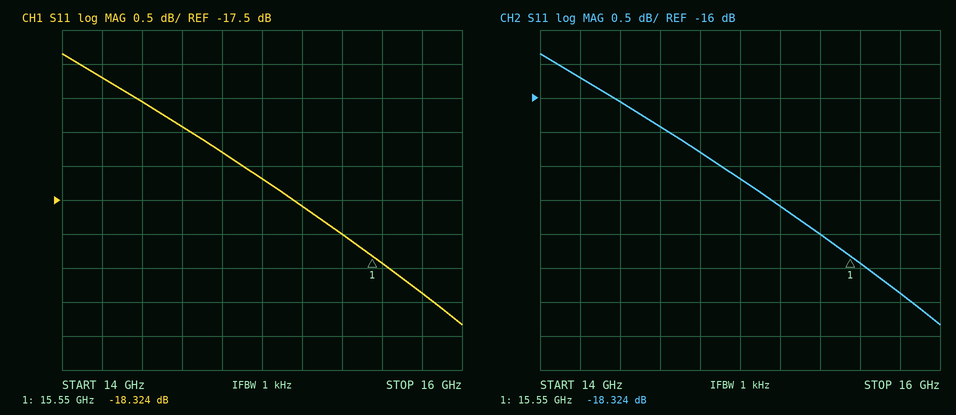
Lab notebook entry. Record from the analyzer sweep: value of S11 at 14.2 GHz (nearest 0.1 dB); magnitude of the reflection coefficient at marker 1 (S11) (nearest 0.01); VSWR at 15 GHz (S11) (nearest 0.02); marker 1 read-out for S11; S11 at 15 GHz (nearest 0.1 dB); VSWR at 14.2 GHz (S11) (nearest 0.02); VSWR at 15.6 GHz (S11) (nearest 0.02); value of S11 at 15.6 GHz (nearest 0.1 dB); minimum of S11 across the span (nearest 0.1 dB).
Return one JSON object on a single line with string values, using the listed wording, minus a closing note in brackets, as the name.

{"value of S11 at 14.2 GHz": "-15.7 dB", "magnitude of the reflection coefficient at marker 1 (S11)": "0.12", "VSWR at 15 GHz (S11)": "1.32", "marker 1 read-out for S11": "-18.324 dB", "S11 at 15 GHz": "-17.2 dB", "VSWR at 14.2 GHz (S11)": "1.40", "VSWR at 15.6 GHz (S11)": "1.28", "value of S11 at 15.6 GHz": "-18.4 dB", "minimum of S11 across the span": "-19.3 dB"}
